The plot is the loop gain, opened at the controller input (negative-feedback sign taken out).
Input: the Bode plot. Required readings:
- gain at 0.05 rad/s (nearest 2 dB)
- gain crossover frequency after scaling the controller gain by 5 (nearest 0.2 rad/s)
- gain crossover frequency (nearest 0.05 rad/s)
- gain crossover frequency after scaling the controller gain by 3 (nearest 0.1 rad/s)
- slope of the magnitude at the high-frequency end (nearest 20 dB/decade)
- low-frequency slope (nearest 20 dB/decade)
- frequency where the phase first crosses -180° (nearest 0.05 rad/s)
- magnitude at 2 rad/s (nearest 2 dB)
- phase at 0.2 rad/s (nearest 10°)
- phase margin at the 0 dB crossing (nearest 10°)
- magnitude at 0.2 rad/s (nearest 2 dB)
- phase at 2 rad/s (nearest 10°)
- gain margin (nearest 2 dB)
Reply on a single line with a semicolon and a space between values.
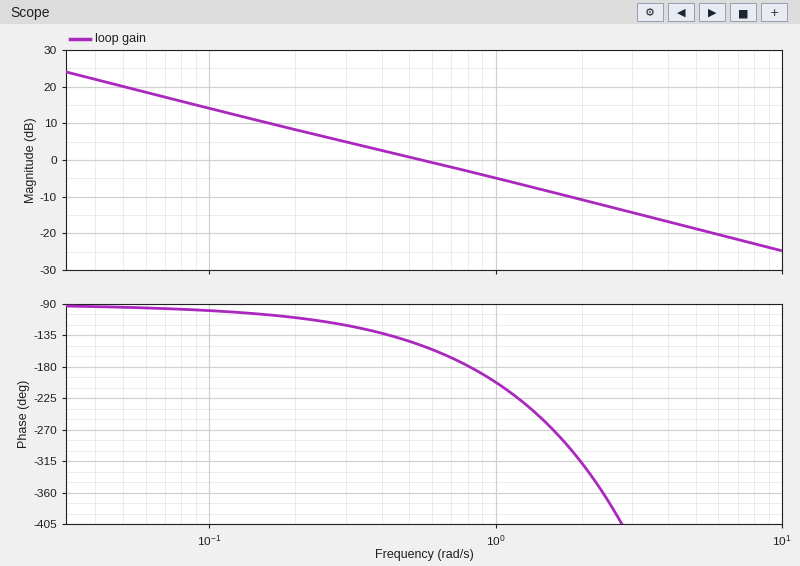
20 dB; 2.8 rad/s; 0.55 rad/s; 1.7 rad/s; -20 dB/decade; -20 dB/decade; 0.80 rad/s; -10 dB; -110°; 30°; 8 dB; -320°; 4 dB
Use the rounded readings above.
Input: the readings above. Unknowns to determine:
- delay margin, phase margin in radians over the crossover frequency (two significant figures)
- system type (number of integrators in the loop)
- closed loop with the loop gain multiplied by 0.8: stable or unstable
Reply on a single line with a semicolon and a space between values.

0.95 s; 1; stable
